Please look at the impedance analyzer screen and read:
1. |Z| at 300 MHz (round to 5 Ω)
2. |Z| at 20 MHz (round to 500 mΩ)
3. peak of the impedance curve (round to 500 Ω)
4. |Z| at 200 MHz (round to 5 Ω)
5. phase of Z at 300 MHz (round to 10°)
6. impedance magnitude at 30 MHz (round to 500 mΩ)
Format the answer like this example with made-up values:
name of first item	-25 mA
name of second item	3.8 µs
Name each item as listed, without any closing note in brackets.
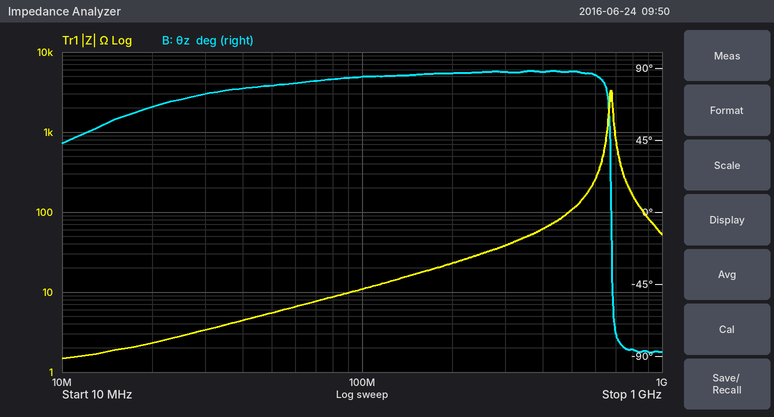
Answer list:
|Z| at 300 MHz	40 Ω
|Z| at 20 MHz	2.5 Ω
peak of the impedance curve	3.5 kΩ
|Z| at 200 MHz	25 Ω
phase of Z at 300 MHz	90°
impedance magnitude at 30 MHz	3.5 Ω
